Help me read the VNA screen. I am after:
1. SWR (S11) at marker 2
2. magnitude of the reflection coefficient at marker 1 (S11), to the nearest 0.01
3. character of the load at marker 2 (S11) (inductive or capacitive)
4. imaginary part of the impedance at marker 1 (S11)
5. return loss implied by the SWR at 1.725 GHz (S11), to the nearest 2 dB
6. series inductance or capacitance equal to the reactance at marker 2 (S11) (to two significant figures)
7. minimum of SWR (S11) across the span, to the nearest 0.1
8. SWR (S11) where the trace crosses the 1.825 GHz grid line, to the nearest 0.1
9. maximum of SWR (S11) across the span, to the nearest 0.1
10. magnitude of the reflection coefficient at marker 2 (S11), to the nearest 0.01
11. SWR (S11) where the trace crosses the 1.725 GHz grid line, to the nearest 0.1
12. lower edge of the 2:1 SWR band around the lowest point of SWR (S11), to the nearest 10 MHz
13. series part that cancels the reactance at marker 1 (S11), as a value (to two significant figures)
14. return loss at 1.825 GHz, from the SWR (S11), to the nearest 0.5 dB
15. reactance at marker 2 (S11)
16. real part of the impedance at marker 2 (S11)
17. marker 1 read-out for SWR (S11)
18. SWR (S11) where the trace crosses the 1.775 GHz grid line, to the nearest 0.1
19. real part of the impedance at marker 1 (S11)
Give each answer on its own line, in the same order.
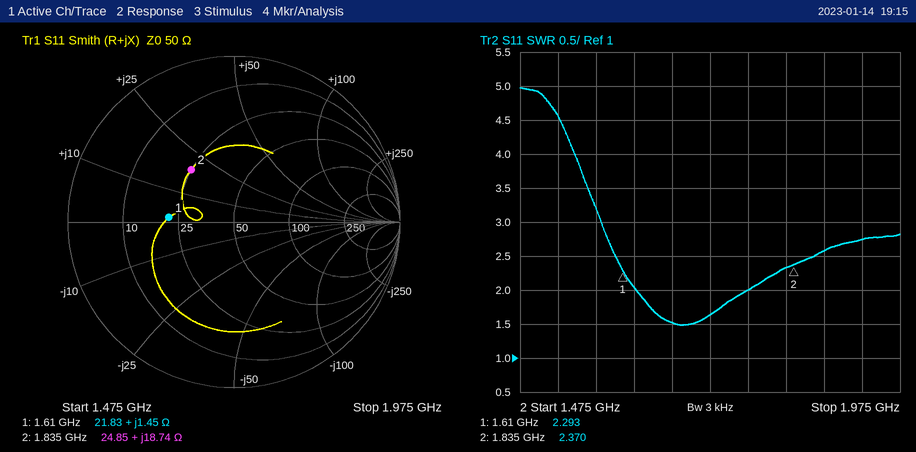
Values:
2.370
0.39
inductive
+1.45 Ω
12 dB
1.6 nH
1.5
2.3
5.0
0.41
1.6
1.63 GHz
68 pF
8.0 dB
+18.74 Ω
24.85 Ω
2.293
2.0
21.83 Ω
